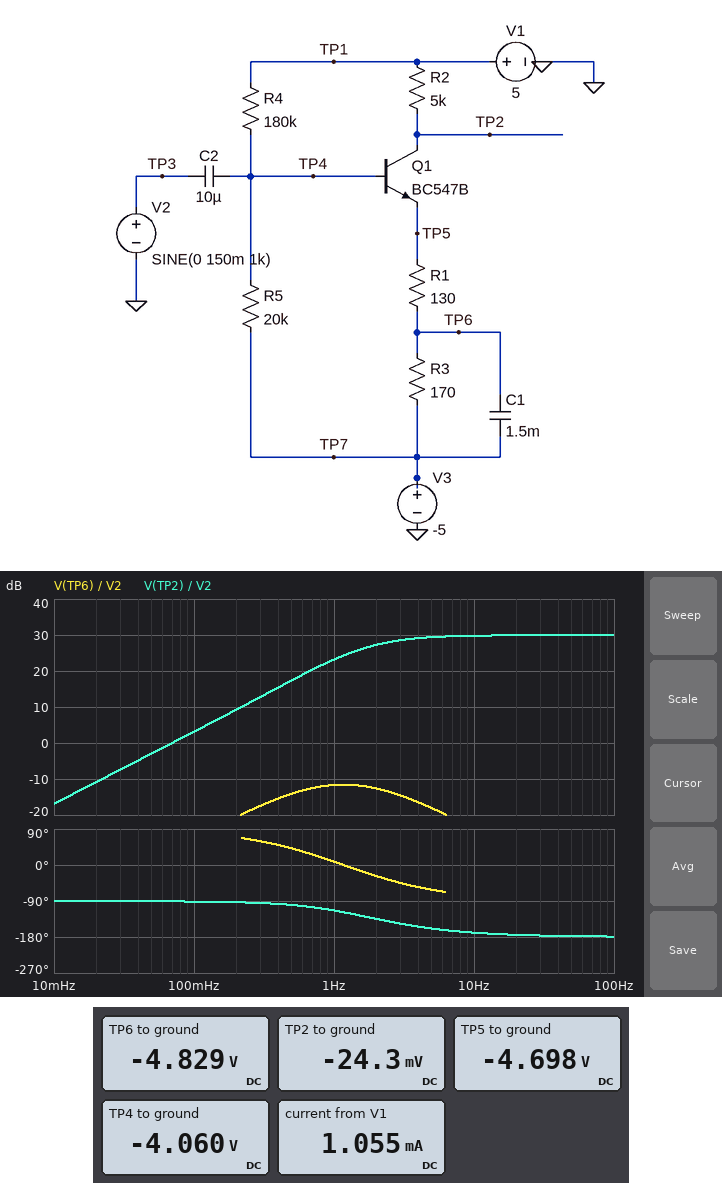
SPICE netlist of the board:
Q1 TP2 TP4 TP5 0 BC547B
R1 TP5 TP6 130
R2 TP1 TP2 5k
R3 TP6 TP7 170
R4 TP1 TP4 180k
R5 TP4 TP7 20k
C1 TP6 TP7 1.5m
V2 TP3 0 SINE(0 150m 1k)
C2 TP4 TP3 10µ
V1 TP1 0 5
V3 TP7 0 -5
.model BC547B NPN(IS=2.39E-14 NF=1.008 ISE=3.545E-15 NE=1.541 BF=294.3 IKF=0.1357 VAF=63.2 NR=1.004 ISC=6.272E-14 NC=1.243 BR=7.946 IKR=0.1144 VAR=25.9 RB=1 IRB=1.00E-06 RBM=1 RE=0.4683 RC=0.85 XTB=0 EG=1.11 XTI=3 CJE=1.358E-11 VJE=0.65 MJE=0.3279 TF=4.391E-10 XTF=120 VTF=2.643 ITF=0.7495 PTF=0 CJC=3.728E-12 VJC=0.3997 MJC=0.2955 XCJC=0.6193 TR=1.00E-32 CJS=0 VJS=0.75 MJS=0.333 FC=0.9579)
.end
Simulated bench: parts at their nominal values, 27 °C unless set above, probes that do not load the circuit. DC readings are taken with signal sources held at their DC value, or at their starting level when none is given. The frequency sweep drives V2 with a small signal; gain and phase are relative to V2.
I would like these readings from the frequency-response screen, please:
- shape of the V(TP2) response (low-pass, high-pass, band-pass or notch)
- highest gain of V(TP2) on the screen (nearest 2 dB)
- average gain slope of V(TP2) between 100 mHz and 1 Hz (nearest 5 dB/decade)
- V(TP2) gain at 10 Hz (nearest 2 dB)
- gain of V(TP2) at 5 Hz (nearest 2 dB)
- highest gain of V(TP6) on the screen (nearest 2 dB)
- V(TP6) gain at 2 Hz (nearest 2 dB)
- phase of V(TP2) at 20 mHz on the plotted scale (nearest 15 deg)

high-pass
30 dB
20 dB/decade
30 dB
30 dB
-12 dB
-12 dB
-90 deg
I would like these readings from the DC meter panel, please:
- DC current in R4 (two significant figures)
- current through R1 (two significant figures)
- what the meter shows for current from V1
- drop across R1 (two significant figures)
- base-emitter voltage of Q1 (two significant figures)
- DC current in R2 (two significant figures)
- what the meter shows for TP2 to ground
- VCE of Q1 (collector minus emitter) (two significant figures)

50 µA
1.0 mA
1.055 mA
130 mV
640 mV
1.0 mA
-24.3 mV
4.7 V
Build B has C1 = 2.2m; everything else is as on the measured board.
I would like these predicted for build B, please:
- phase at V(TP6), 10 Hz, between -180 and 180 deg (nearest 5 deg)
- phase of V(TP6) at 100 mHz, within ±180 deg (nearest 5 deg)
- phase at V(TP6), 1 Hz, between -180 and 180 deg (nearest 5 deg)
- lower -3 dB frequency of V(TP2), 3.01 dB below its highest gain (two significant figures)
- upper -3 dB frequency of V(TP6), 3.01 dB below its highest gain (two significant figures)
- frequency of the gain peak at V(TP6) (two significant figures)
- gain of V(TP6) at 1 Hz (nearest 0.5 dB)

-80 deg
75 deg
0 deg
1.6 Hz
2.5 Hz
970 mHz
-13.5 dB
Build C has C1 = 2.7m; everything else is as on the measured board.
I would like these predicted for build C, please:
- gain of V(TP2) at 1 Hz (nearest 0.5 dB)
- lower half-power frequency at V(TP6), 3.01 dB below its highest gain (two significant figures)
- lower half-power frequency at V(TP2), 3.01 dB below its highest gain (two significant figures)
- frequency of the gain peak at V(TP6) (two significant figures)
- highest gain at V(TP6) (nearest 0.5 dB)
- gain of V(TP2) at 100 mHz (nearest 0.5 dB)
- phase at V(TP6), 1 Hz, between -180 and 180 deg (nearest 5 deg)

24.5 dB
330 mHz
1.5 Hz
870 mHz
-14.5 dB
3.5 dB
-5 deg
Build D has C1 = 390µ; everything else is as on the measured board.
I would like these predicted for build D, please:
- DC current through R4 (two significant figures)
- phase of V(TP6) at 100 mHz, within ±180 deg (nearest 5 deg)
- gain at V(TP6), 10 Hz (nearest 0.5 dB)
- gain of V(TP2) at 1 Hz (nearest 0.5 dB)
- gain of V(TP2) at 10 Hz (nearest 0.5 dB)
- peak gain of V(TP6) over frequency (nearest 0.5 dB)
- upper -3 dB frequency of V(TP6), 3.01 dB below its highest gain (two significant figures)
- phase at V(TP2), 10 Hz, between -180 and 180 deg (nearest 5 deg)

50 µA
85 deg
-13.0 dB
20.5 dB
29.0 dB
-7.5 dB
7.0 Hz
-160 deg
